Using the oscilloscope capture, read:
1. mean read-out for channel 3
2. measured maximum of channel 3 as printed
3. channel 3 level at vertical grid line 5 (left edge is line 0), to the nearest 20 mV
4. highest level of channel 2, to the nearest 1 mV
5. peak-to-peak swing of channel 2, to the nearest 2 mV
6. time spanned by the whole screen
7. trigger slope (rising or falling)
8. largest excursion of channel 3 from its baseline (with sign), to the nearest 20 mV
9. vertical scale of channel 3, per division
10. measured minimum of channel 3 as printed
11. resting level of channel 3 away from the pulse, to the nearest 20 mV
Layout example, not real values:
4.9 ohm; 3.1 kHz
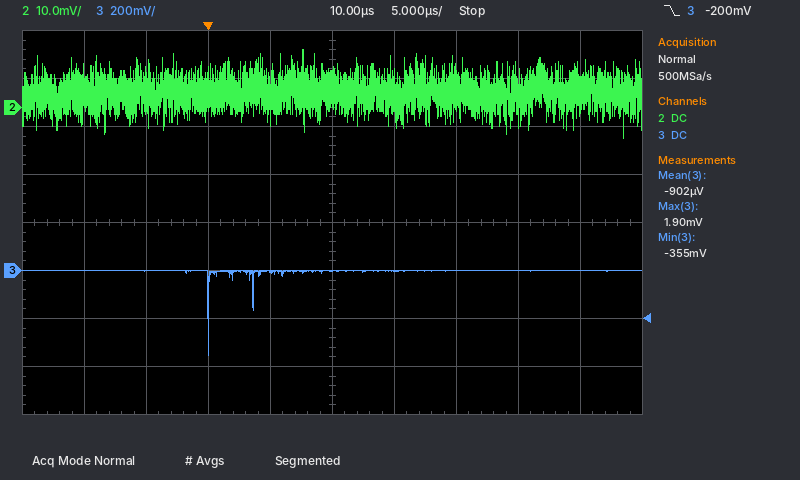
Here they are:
-902 µV; 1.90 mV; 0 mV; 12 mV; 18 mV; 50 µs; falling; -360 mV; 200 mV; -355 mV; 0 mV
